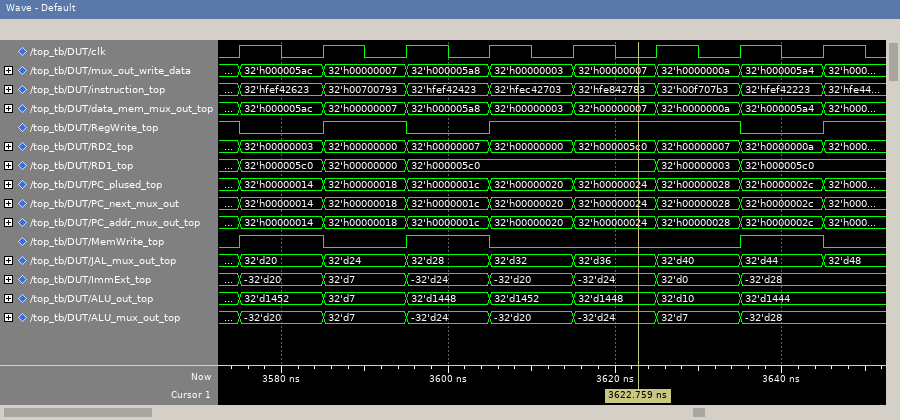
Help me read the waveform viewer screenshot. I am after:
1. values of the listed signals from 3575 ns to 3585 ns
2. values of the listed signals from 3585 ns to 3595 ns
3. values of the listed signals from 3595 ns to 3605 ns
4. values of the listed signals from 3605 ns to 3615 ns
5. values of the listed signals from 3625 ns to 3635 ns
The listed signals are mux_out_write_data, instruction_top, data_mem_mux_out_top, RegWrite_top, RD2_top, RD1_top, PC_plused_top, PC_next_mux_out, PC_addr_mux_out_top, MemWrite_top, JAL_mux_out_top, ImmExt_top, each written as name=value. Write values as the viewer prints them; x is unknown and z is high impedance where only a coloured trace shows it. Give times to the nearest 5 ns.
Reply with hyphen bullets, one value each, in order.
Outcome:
- mux_out_write_data=32'h000005ac, instruction_top=32'hfef42623, data_mem_mux_out_top=32'h000005ac, RegWrite_top=0, RD2_top=32'h00000003, RD1_top=32'h000005c0, PC_plused_top=32'h00000014, PC_next_mux_out=32'h00000014, PC_addr_mux_out_top=32'h00000014, MemWrite_top=1, JAL_mux_out_top=32'd20, ImmExt_top=-32'd20
- mux_out_write_data=32'h00000007, instruction_top=32'h00700793, data_mem_mux_out_top=32'h00000007, RegWrite_top=1, RD2_top=32'h00000000, RD1_top=32'h00000000, PC_plused_top=32'h00000018, PC_next_mux_out=32'h00000018, PC_addr_mux_out_top=32'h00000018, MemWrite_top=0, JAL_mux_out_top=32'd24, ImmExt_top=32'd7
- mux_out_write_data=32'h000005a8, instruction_top=32'hfef42423, data_mem_mux_out_top=32'h000005a8, RegWrite_top=0, RD2_top=32'h00000007, RD1_top=32'h000005c0, PC_plused_top=32'h0000001c, PC_next_mux_out=32'h0000001c, PC_addr_mux_out_top=32'h0000001c, MemWrite_top=1, JAL_mux_out_top=32'd28, ImmExt_top=-32'd24
- mux_out_write_data=32'h00000003, instruction_top=32'hfec42703, data_mem_mux_out_top=32'h00000003, RegWrite_top=1, RD2_top=32'h00000000, RD1_top=32'h000005c0, PC_plused_top=32'h00000020, PC_next_mux_out=32'h00000020, PC_addr_mux_out_top=32'h00000020, MemWrite_top=0, JAL_mux_out_top=32'd32, ImmExt_top=-32'd20
- mux_out_write_data=32'h0000000a, instruction_top=32'h00f707b3, data_mem_mux_out_top=32'h0000000a, RegWrite_top=1, RD2_top=32'h00000007, RD1_top=32'h00000003, PC_plused_top=32'h00000028, PC_next_mux_out=32'h00000028, PC_addr_mux_out_top=32'h00000028, MemWrite_top=0, JAL_mux_out_top=32'd40, ImmExt_top=32'd0
